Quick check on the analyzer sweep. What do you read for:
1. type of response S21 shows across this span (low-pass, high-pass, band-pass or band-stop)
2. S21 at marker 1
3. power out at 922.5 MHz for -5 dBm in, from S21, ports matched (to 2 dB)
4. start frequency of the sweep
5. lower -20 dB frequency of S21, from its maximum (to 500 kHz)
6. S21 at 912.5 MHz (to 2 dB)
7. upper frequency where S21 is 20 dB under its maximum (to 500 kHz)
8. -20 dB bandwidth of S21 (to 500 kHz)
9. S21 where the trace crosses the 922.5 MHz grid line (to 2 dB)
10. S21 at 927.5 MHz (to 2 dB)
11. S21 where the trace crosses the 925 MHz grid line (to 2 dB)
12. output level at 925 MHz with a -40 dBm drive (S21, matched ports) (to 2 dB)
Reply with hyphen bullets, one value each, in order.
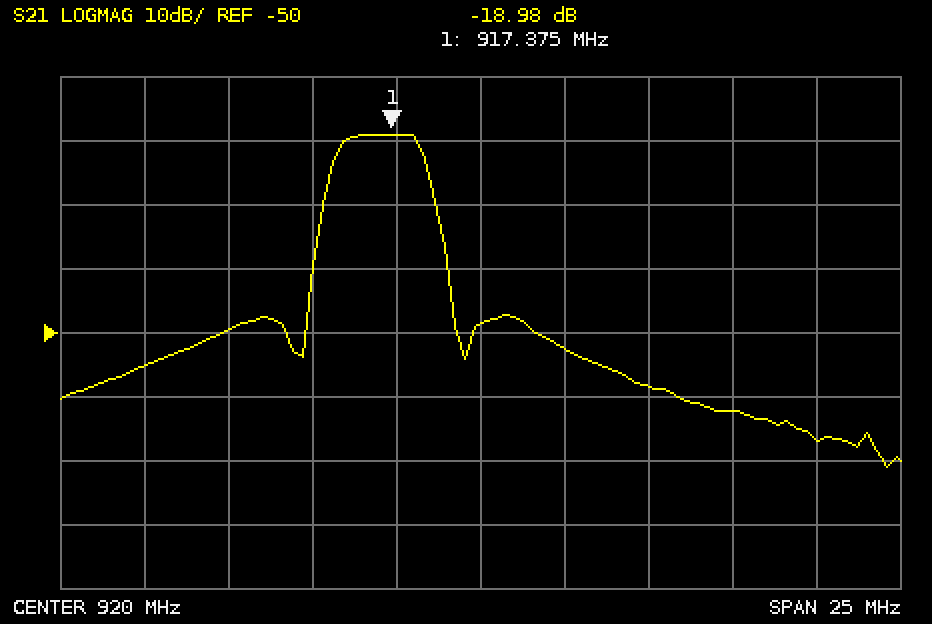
- band-pass
- -18.98 dB
- -58 dBm
- 907.5 MHz
- 915.0 MHz
- -50 dB
- 919.0 MHz
- 4.0 MHz
- -52 dB
- -62 dB
- -58 dB
- -98 dBm
